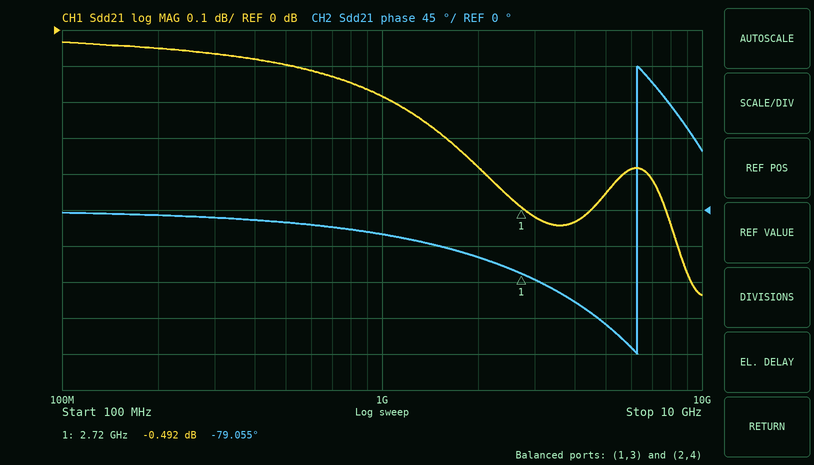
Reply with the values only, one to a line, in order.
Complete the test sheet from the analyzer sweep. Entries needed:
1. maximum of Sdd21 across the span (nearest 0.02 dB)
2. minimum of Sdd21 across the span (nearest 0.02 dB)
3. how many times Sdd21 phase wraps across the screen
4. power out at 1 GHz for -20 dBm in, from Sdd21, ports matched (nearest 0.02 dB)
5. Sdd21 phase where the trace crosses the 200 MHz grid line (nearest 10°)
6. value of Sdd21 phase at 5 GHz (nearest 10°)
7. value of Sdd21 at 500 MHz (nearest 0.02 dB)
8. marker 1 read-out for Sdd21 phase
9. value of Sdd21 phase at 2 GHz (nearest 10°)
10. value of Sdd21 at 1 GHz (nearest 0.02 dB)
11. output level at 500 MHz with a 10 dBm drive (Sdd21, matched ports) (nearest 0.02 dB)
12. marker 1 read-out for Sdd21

-0.04 dB
-0.74 dB
1
-20.18 dBm
-10°
-140°
-0.10 dB
-79.055°
-60°
-0.18 dB
9.90 dBm
-0.492 dB
